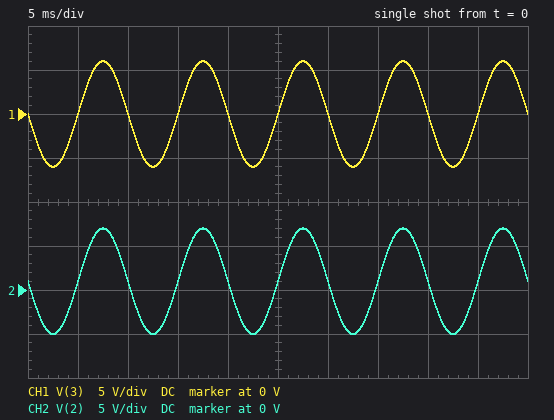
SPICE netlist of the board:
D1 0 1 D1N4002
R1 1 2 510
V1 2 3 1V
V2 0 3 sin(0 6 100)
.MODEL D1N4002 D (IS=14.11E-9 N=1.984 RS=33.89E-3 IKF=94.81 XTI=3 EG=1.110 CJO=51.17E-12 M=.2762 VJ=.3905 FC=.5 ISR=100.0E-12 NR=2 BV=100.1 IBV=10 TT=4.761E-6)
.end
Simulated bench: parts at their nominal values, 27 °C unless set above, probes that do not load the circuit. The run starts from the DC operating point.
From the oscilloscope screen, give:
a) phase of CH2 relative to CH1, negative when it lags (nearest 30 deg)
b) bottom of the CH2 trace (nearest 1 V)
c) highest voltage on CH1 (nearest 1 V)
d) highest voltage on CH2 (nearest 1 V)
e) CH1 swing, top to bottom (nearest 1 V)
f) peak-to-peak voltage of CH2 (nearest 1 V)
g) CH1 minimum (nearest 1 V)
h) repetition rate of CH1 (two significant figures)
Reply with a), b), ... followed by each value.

a) 0 deg
b) -5 V
c) 6 V
d) 7 V
e) 12 V
f) 12 V
g) -6 V
h) 100 Hz
